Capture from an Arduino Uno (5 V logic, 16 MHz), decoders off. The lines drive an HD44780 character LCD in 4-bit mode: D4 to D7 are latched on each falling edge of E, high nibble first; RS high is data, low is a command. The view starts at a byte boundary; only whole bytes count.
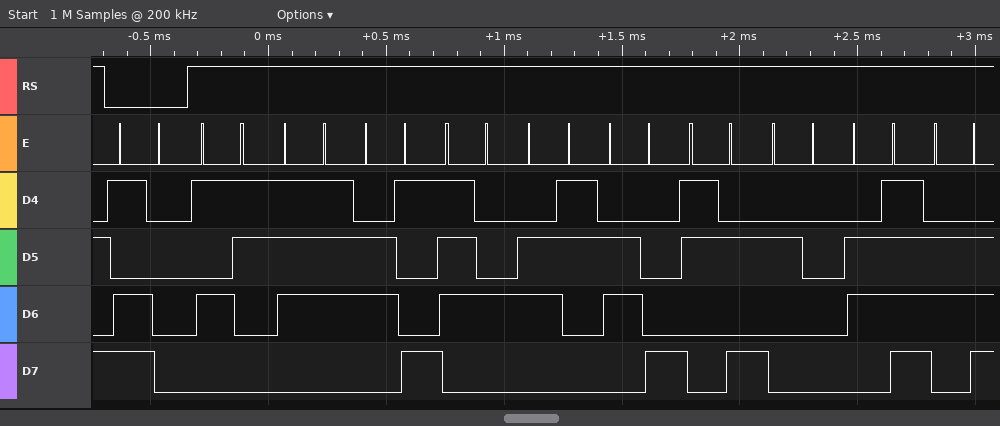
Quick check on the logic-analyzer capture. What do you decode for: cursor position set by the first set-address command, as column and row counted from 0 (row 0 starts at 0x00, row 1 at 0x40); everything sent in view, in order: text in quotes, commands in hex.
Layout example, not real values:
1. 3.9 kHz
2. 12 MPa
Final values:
1. column 16, row 1
2. 0xD0 "Switch: on"
